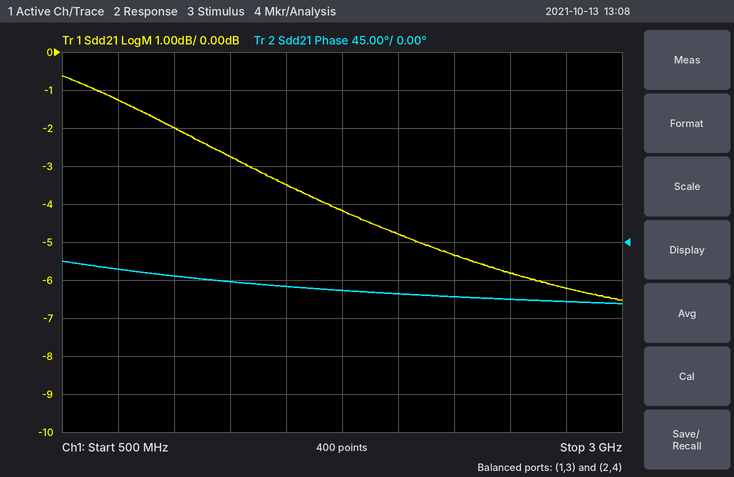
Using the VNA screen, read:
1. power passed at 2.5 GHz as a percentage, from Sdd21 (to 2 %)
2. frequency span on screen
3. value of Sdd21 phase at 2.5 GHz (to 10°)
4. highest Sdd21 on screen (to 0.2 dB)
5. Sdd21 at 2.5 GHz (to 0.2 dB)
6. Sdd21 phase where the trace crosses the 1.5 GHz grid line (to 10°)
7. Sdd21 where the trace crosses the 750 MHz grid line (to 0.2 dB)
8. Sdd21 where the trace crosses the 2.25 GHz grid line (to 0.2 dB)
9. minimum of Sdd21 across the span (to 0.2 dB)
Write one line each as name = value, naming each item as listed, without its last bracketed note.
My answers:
power passed at 2.5 GHz as a percentage, from Sdd21 = 26 %
frequency span on screen = 2.5 GHz
value of Sdd21 phase at 2.5 GHz = -70°
highest Sdd21 on screen = -0.6 dB
Sdd21 at 2.5 GHz = -5.8 dB
Sdd21 phase where the trace crosses the 1.5 GHz grid line = -50°
Sdd21 where the trace crosses the 750 MHz grid line = -1.2 dB
Sdd21 where the trace crosses the 2.25 GHz grid line = -5.4 dB
minimum of Sdd21 across the span = -6.6 dB
